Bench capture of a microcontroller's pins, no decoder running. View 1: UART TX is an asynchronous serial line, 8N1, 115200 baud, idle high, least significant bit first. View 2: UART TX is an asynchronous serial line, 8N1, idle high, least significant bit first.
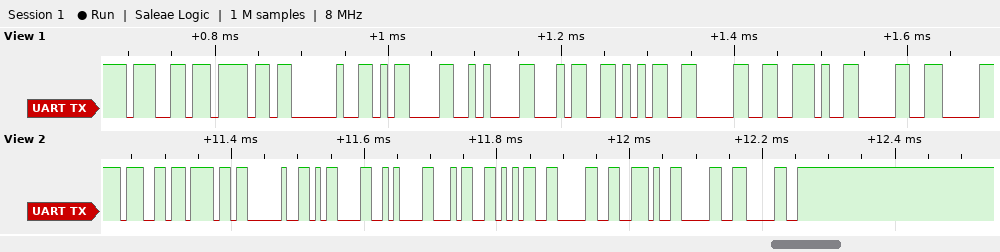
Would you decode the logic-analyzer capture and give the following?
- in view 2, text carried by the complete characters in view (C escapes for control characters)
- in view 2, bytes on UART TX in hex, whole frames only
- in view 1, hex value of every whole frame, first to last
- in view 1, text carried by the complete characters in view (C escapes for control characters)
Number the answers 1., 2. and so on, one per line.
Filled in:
1. "go \r\n450.00"
2. 67 6F 20 0D 0A 34 35 30 2E 30 30
3. 0x67 0x6F 0x20 0x0D 0x0A 0x34 0x35 0x30 0x2E 0x30
4. "go \r\n450.0"
